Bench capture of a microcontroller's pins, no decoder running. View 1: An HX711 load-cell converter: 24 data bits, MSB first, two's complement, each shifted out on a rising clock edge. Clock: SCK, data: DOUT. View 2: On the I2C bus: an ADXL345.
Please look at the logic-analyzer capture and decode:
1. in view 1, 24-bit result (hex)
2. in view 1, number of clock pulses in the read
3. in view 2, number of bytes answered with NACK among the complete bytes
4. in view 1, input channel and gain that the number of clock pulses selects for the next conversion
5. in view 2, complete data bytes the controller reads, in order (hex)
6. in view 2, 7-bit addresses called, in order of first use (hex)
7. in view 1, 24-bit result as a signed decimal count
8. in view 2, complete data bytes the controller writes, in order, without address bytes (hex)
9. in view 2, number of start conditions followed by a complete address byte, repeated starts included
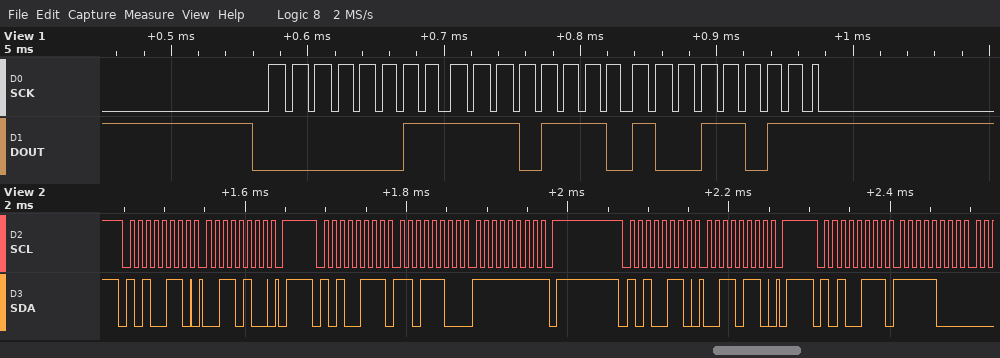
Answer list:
0x03EE9B
25
1
channel A, gain 128
DC FF F8
0x53
257691
34 36
4
